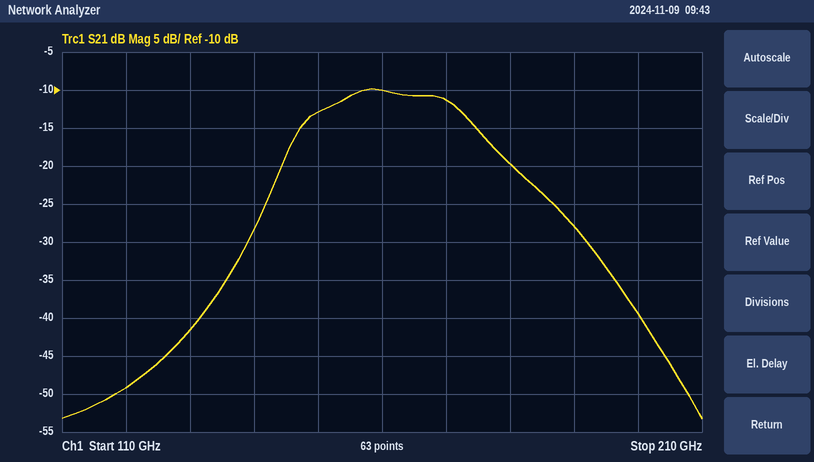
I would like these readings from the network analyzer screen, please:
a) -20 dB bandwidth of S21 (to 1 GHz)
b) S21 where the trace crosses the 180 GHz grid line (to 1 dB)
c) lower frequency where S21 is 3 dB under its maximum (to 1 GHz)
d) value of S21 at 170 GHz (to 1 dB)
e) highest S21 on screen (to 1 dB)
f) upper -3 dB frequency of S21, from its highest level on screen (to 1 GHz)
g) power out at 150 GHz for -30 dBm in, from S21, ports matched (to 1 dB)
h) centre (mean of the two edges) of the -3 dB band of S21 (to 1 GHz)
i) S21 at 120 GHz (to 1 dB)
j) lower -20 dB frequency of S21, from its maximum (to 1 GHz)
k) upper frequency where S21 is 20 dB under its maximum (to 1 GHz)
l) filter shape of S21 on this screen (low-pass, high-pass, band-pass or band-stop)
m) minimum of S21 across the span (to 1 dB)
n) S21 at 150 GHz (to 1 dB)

53 GHz
-20 dB
150 GHz
-11 dB
-10 dB
172 GHz
-43 dBm
161 GHz
-49 dB
139 GHz
192 GHz
band-pass
-53 dB
-13 dB
